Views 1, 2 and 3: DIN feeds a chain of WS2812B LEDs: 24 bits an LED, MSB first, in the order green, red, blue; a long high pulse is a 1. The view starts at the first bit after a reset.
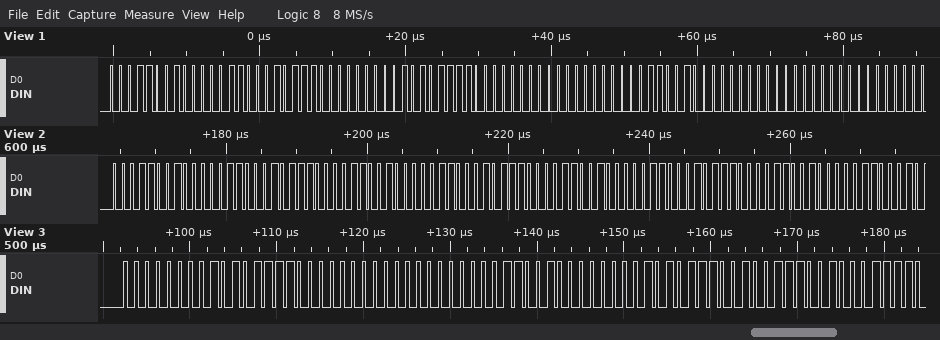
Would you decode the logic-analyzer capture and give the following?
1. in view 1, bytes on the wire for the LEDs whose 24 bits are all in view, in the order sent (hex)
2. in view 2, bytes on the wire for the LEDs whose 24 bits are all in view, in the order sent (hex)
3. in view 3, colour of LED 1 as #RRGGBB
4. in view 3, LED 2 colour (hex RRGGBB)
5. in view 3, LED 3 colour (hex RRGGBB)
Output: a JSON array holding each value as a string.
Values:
["19 06 2E 00 AF 00 00 19 00", "19 06 2E 19 06 2E 19 06 2E", "#AF0000", "#190000", "#4EAE47"]
